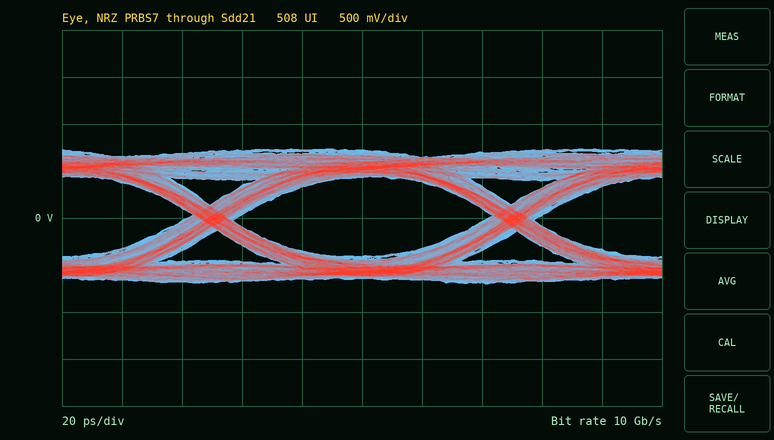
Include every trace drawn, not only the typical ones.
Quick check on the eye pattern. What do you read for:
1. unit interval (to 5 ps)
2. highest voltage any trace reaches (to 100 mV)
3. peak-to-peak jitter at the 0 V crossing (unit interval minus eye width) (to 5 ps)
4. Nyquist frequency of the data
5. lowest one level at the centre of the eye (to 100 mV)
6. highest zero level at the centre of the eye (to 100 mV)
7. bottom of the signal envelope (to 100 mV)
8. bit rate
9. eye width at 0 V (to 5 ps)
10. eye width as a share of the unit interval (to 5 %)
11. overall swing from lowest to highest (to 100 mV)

100 ps
700 mV
15 ps
5 GHz
400 mV
-400 mV
-700 mV
10 Gb/s
85 ps
85 %
1.4 V
